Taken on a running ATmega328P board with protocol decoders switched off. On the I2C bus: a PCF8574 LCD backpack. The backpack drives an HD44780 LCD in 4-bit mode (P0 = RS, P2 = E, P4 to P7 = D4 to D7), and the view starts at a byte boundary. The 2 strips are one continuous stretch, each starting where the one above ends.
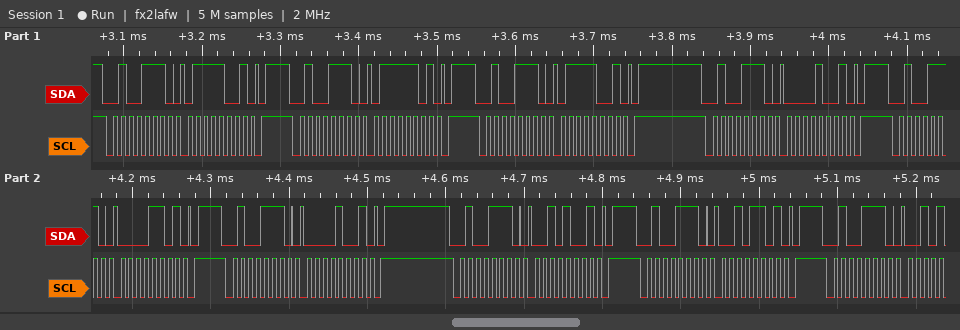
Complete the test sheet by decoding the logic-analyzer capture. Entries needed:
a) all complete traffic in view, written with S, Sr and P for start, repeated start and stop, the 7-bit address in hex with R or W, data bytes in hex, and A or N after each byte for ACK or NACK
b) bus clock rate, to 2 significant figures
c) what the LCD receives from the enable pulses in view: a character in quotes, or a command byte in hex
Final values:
S 27W A 79 A P S 27W A 7D A P S 27W A 79 A P S 27W A 09 A P S 27W A 0D A P S 27W A 09 A P S 27W A 29 A P S 27W A 2D A P S 27W A
100 kHz
'p'
